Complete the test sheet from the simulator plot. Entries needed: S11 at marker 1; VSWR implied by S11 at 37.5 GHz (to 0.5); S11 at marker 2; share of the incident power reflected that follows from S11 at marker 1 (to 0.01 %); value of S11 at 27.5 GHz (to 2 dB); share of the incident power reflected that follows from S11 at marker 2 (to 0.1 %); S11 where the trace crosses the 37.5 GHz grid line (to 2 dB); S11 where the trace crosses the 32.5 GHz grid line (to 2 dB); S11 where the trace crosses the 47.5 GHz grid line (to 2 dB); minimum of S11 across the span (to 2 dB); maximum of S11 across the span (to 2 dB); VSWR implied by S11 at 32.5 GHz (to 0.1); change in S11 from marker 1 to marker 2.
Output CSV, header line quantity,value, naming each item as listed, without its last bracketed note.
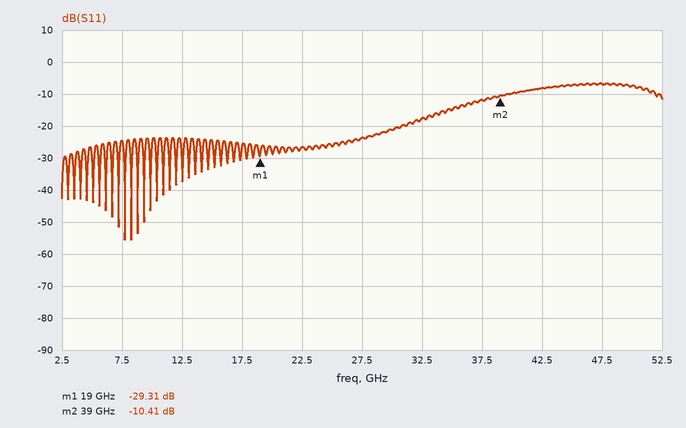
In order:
quantity,value
S11 at marker 1,-29.31 dB
VSWR implied by S11 at 37.5 GHz,1.5
S11 at marker 2,-10.41 dB
share of the incident power reflected that follows from S11 at marker 1,0.12 %
value of S11 at 27.5 GHz,-24 dB
share of the incident power reflected that follows from S11 at marker 2,9.1 %
S11 where the trace crosses the 37.5 GHz grid line,-12 dB
S11 where the trace crosses the 32.5 GHz grid line,-18 dB
S11 where the trace crosses the 47.5 GHz grid line,-6 dB
minimum of S11 across the span,-56 dB
maximum of S11 across the span,-6 dB
VSWR implied by S11 at 32.5 GHz,1.3
change in S11 from marker 1 to marker 2,18.90 dB
